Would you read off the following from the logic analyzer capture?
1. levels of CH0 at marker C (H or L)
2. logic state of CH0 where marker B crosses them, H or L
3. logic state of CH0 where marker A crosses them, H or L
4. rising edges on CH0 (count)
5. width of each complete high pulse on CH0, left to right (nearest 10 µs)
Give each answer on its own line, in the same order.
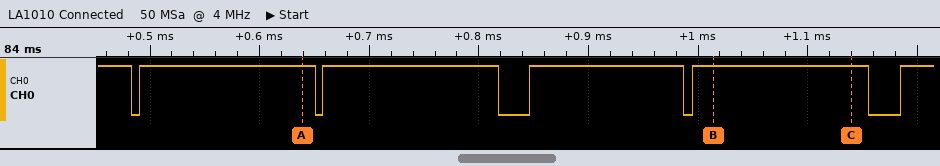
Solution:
CH0=H
CH0=H
CH0=H
5
160 µs, 160 µs, 140 µs, 160 µs
